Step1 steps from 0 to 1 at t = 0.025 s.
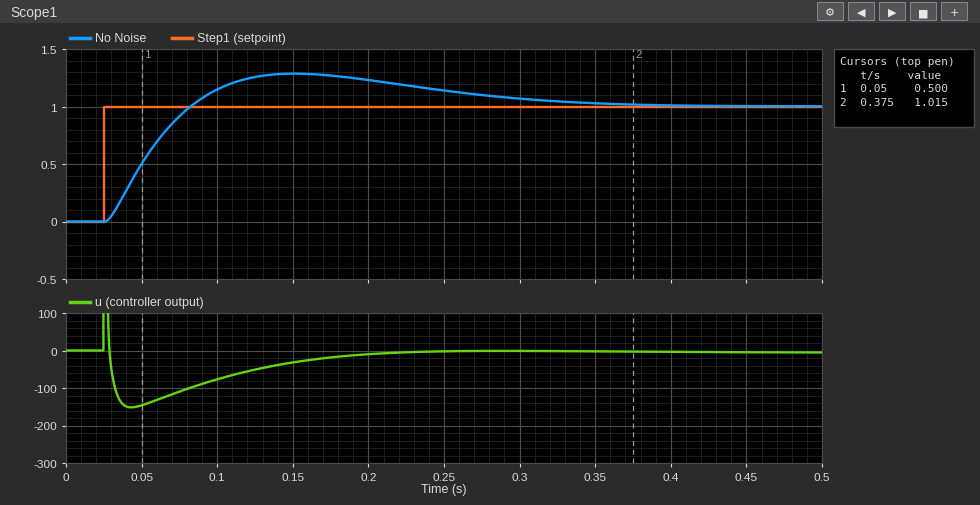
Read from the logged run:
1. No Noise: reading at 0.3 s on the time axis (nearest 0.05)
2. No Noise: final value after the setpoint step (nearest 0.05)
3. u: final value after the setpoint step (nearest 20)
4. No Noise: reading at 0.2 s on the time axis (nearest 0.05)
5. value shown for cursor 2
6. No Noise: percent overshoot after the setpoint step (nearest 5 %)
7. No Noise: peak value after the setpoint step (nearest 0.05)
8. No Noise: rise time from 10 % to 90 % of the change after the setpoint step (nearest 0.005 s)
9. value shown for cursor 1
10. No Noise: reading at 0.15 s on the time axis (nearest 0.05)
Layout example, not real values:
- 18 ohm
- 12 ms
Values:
- 1.05
- 1.00
- 0
- 1.25
- 1.015
- 30 %
- 1.30
- 0.040 s
- 0.500
- 1.30
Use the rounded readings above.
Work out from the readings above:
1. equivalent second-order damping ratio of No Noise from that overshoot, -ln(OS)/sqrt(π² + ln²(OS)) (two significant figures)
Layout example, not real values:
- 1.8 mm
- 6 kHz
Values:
- 0.36
